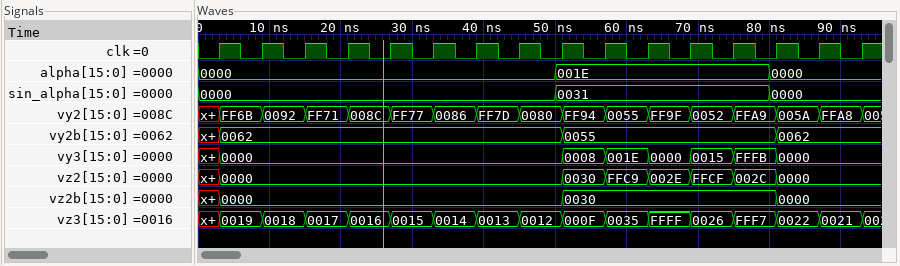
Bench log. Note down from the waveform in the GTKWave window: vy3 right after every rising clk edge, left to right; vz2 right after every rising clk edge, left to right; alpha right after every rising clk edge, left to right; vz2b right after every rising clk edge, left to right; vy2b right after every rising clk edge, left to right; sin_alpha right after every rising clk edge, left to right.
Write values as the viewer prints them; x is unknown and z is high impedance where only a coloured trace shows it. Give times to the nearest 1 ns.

0000, 0000, 0000, 0000, 0000, 0000, 0000, 0000, 0008, 001E, 0000, 0015, FFFB, 0000, 0000, 0000
0000, 0000, 0000, 0000, 0000, 0000, 0000, 0000, 0030, FFC9, 002E, FFCF, 002C, 0000, 0000, 0000
0000, 0000, 0000, 0000, 0000, 0000, 0000, 0000, 001E, 001E, 001E, 001E, 001E, 0000, 0000, 0000
0000, 0000, 0000, 0000, 0000, 0000, 0000, 0000, 0030, 0030, 0030, 0030, 0030, 0000, 0000, 0000
0062, 0062, 0062, 0062, 0062, 0062, 0062, 0062, 0055, 0055, 0055, 0055, 0055, 0062, 0062, 0062
0000, 0000, 0000, 0000, 0000, 0000, 0000, 0000, 0031, 0031, 0031, 0031, 0031, 0000, 0000, 0000
